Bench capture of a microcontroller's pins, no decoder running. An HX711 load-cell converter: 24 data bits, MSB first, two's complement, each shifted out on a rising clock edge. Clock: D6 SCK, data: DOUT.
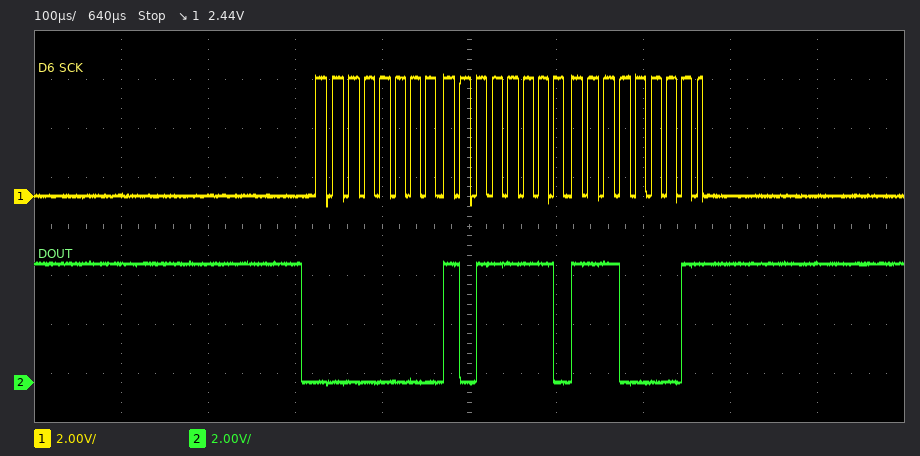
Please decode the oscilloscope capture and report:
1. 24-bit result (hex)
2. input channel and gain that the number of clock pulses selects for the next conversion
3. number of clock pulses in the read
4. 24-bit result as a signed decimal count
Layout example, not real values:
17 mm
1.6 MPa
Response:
0x00BEE1
channel A, gain 128
25
48865
